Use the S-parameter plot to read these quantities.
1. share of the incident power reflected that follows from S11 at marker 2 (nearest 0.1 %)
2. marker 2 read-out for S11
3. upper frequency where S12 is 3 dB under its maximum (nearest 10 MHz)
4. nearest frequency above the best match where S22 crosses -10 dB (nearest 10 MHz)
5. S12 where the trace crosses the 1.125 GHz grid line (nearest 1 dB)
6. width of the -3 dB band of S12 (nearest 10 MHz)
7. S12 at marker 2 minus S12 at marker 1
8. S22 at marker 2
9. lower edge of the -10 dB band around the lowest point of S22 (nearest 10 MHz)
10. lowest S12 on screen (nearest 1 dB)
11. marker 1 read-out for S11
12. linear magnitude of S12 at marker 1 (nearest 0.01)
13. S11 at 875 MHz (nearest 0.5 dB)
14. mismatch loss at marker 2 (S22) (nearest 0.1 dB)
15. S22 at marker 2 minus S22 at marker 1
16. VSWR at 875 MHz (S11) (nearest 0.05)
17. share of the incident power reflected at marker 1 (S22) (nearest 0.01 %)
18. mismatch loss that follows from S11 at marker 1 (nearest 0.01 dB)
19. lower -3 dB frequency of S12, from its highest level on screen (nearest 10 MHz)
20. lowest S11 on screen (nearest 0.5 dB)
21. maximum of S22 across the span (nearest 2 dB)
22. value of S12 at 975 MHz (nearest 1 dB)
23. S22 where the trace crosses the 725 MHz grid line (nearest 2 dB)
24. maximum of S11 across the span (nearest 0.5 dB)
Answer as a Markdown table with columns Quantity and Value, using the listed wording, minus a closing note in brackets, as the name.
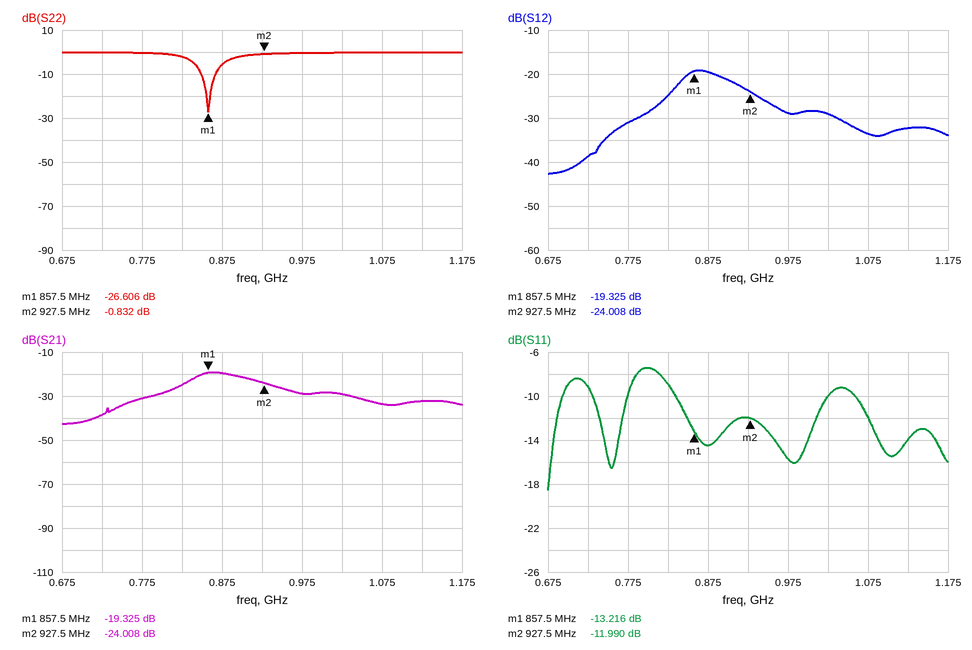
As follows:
| Quantity | Value |
|---|---|
| share of the incident power reflected that follows from S11 at marker 2 | 6.3 % |
| marker 2 read-out for S11 | -11.990 dB |
| upper frequency where S12 is 3 dB under its maximum | 910 MHz |
| nearest frequency above the best match where S22 crosses -10 dB | 870 MHz |
| S12 where the trace crosses the 1.125 GHz grid line | -32 dB |
| width of the -3 dB band of S12 | 70 MHz |
| S12 at marker 2 minus S12 at marker 1 | -4.683 dB |
| S22 at marker 2 | -0.832 dB |
| lower edge of the -10 dB band around the lowest point of S22 | 850 MHz |
| lowest S12 on screen | -43 dB |
| marker 1 read-out for S11 | -13.216 dB |
| linear magnitude of S12 at marker 1 | 0.11 |
| S11 at 875 MHz | -14.5 dB |
| mismatch loss at marker 2 (S22) | 7.6 dB |
| S22 at marker 2 minus S22 at marker 1 | 25.774 dB |
| VSWR at 875 MHz (S11) | 1.45 |
| share of the incident power reflected at marker 1 (S22) | 0.22 % |
| mismatch loss that follows from S11 at marker 1 | 0.21 dB |
| lower -3 dB frequency of S12, from its highest level on screen | 840 MHz |
| lowest S11 on screen | -18.5 dB |
| maximum of S22 across the span | 0 dB |
| value of S12 at 975 MHz | -29 dB |
| S22 where the trace crosses the 725 MHz grid line | 0 dB |
| maximum of S11 across the span | -7.5 dB |
